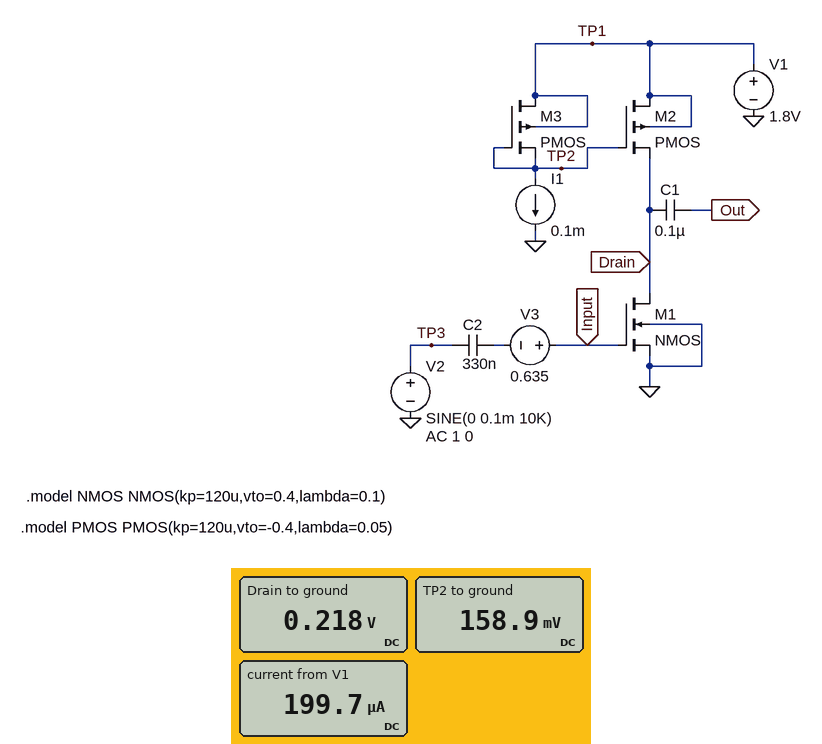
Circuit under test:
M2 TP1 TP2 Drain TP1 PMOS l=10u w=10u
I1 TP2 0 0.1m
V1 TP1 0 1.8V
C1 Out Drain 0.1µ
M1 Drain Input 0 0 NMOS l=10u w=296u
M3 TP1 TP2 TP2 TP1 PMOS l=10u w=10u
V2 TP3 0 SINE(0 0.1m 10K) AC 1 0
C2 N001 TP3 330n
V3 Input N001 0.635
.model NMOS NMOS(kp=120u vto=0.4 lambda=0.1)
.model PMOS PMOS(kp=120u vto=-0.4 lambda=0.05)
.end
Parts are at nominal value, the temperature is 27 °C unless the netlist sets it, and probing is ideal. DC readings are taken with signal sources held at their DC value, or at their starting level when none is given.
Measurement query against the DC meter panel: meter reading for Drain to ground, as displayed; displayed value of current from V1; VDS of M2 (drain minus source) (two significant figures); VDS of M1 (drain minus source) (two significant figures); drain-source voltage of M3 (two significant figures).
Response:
0.218 V
199.7 µA
1.6 V
220 mV
1.6 V
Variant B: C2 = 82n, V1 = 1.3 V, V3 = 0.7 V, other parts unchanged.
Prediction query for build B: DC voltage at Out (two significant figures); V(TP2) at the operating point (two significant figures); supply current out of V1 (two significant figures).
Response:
110 mV
-340 mV
200 µA
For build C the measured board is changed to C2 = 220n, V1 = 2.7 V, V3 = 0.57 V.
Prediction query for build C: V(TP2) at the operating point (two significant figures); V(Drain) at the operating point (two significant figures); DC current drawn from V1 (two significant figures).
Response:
1.1 V
2.2 V
160 µA
